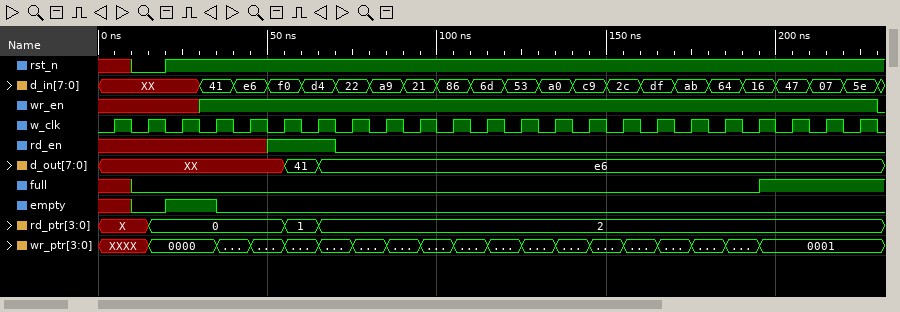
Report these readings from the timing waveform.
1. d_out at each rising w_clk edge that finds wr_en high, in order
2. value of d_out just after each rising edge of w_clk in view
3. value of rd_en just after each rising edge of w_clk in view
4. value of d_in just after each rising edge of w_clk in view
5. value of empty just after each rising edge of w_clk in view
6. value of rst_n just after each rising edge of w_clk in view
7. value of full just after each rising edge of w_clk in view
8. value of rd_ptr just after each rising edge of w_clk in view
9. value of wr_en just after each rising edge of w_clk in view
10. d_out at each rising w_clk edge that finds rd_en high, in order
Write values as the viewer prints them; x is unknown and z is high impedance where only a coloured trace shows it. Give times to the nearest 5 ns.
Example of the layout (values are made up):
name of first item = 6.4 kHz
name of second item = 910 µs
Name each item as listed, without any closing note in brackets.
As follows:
d_out at each rising w_clk edge that finds wr_en high, in order = XX, XX, XX, 41, e6, e6, e6, e6, e6, e6, e6, e6, e6, e6, e6, e6, e6, e6, e6, e6
value of d_out just after each rising edge of w_clk in view = XX, XX, XX, XX, XX, 41, e6, e6, e6, e6, e6, e6, e6, e6, e6, e6, e6, e6, e6, e6, e6, e6, e6
value of rd_en just after each rising edge of w_clk in view = x x x x x 1 1 0 0 0 0 0 0 0 0 0 0 0 0 0 0 0 0
value of d_in just after each rising edge of w_clk in view = XX, XX, XX, 41, e6, f0, d4, 22, a9, 21, 86, 6d, 53, a0, c9, 2c, df, ab, 64, 16, 47, 07, 5e
value of empty just after each rising edge of w_clk in view = x 0 1 0 0 0 0 0 0 0 0 0 0 0 0 0 0 0 0 0 0 0 0
value of rst_n just after each rising edge of w_clk in view = x 0 1 1 1 1 1 1 1 1 1 1 1 1 1 1 1 1 1 1 1 1 1
value of full just after each rising edge of w_clk in view = x 0 0 0 0 0 0 0 0 0 0 0 0 0 0 0 0 0 0 1 1 1 1
value of rd_ptr just after each rising edge of w_clk in view = X, 0, 0, 0, 0, 1, 2, 2, 2, 2, 2, 2, 2, 2, 2, 2, 2, 2, 2, 2, 2, 2, 2
value of wr_en just after each rising edge of w_clk in view = x x x 1 1 1 1 1 1 1 1 1 1 1 1 1 1 1 1 1 1 1 1
d_out at each rising w_clk edge that finds rd_en high, in order = XX, 41
